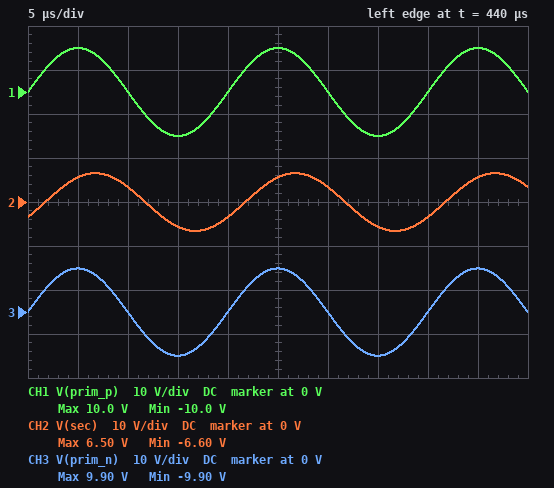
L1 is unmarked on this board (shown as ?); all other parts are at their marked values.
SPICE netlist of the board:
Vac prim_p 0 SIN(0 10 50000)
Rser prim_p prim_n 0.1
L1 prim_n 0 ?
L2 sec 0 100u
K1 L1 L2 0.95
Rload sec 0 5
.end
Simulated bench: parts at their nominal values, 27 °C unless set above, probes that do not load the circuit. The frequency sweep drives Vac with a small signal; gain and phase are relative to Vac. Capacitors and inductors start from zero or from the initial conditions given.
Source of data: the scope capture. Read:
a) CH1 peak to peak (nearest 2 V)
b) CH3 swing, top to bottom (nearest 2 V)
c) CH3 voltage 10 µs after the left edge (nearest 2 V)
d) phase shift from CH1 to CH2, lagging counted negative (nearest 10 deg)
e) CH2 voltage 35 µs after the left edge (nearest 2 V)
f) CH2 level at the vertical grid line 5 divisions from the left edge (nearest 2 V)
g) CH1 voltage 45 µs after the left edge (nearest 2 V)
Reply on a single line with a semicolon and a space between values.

20 V; 20 V; 0 V; -30 deg; -6 V; 6 V; 10 V
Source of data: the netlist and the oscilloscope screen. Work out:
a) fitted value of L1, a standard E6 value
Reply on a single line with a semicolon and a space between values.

150 µH
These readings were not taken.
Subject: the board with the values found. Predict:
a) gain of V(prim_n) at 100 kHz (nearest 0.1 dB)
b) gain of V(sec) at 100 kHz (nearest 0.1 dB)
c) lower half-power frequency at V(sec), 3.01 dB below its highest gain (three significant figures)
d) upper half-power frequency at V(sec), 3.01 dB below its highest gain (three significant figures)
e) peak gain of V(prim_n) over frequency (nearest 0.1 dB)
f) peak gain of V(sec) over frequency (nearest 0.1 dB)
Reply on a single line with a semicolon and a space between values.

0 dB; -6.2 dB; 105 Hz; 82.8 kHz; 0 dB; -2.3 dB
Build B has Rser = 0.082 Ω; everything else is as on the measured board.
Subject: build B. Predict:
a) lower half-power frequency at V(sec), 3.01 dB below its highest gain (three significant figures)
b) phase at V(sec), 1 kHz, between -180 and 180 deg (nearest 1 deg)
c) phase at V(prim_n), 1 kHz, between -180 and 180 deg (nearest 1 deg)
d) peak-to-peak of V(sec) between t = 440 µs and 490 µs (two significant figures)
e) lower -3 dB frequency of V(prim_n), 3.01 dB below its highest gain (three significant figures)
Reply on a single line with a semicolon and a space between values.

86.0 Hz; 4 deg; 5 deg; 13 V; 87.9 Hz
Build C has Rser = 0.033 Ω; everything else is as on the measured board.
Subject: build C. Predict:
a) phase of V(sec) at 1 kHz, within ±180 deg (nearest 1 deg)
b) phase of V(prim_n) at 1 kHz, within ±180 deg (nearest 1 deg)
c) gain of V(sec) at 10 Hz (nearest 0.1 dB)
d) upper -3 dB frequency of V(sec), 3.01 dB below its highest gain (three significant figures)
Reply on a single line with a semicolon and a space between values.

1 deg; 2 deg; -13.4 dB; 82.0 kHz
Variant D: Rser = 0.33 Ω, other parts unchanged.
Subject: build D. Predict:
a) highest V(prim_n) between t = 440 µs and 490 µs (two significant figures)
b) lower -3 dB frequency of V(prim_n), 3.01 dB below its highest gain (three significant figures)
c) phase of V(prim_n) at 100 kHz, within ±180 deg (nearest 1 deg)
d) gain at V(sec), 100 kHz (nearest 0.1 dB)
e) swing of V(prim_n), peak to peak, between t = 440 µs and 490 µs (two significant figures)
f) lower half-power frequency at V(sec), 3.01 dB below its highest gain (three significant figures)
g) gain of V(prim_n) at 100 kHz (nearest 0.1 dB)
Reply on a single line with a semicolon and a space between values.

9.7 V; 365 Hz; 1 deg; -6.3 dB; 19 V; 334 Hz; -0.1 dB
